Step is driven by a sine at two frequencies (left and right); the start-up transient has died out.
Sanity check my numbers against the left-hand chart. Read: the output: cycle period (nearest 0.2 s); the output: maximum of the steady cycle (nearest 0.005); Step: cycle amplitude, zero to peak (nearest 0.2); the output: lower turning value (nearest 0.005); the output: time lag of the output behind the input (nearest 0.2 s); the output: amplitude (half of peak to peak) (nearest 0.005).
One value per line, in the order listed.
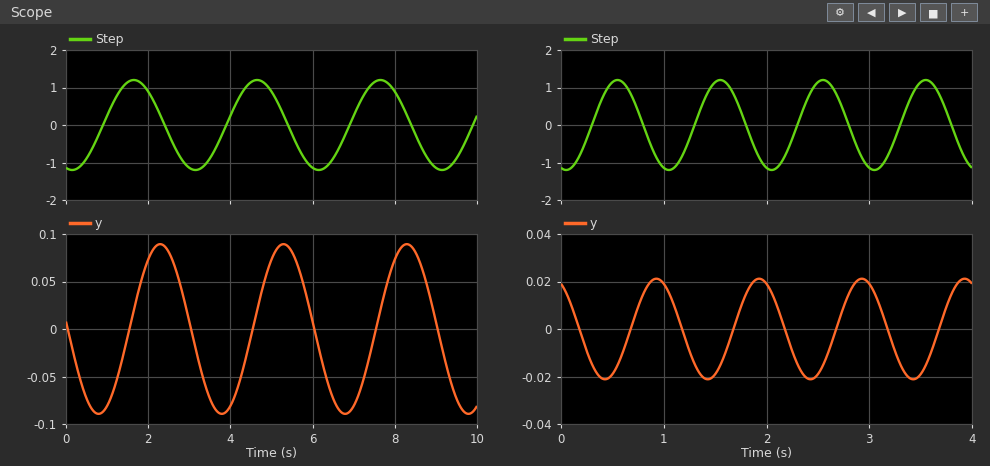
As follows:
3.0 s
0.090
1.2
-0.090
0.6 s
0.090
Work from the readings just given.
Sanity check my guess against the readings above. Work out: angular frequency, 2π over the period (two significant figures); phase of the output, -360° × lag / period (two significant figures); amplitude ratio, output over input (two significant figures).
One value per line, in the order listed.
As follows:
2.1 rad/s
-72°
0.075
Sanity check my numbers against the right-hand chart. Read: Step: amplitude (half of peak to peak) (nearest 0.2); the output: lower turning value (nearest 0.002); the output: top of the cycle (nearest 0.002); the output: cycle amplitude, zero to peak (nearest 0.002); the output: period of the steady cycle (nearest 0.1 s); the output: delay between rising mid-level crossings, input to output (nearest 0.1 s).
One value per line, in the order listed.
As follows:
1.2
-0.022
0.022
0.022
1.0 s
0.4 s
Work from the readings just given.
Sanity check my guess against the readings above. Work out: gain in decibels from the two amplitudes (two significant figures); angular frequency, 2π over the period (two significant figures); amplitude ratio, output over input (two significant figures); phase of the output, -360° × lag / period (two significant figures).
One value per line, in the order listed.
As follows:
-35 dB
6.3 rad/s
0.018
-140°
